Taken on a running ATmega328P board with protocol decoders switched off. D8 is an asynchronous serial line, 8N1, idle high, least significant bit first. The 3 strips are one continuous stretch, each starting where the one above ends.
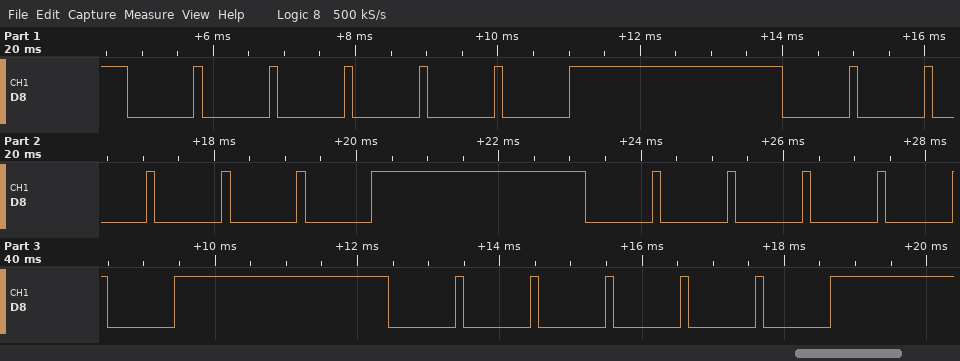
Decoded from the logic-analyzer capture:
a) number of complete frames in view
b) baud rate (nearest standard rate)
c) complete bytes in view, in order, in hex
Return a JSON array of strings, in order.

["24", "9600 baud", "00 00 00 00 00 00 00 00 00 00 00 00 00 00 00 00 00 00 00 00 00 00 00 00"]
